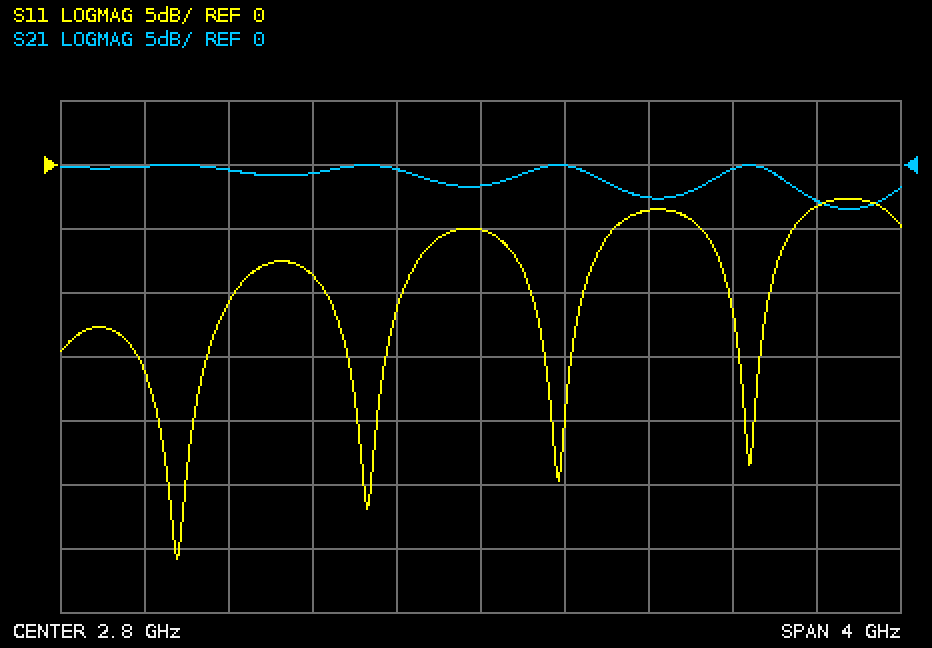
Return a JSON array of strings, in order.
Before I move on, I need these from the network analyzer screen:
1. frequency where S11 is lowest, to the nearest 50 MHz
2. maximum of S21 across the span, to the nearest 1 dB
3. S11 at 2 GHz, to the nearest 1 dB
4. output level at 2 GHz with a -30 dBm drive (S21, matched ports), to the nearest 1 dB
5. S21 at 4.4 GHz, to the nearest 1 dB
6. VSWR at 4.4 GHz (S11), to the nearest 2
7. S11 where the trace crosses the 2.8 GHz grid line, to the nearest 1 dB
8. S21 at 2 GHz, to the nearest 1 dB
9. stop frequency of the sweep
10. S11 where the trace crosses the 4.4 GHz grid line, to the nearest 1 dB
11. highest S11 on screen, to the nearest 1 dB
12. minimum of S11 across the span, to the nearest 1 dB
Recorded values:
["1.35 GHz", "0 dB", "-9 dB", "-31 dBm", "-3 dB", "6", "-5 dB", "-1 dB", "4.8 GHz", "-3 dB", "-3 dB", "-31 dB"]
